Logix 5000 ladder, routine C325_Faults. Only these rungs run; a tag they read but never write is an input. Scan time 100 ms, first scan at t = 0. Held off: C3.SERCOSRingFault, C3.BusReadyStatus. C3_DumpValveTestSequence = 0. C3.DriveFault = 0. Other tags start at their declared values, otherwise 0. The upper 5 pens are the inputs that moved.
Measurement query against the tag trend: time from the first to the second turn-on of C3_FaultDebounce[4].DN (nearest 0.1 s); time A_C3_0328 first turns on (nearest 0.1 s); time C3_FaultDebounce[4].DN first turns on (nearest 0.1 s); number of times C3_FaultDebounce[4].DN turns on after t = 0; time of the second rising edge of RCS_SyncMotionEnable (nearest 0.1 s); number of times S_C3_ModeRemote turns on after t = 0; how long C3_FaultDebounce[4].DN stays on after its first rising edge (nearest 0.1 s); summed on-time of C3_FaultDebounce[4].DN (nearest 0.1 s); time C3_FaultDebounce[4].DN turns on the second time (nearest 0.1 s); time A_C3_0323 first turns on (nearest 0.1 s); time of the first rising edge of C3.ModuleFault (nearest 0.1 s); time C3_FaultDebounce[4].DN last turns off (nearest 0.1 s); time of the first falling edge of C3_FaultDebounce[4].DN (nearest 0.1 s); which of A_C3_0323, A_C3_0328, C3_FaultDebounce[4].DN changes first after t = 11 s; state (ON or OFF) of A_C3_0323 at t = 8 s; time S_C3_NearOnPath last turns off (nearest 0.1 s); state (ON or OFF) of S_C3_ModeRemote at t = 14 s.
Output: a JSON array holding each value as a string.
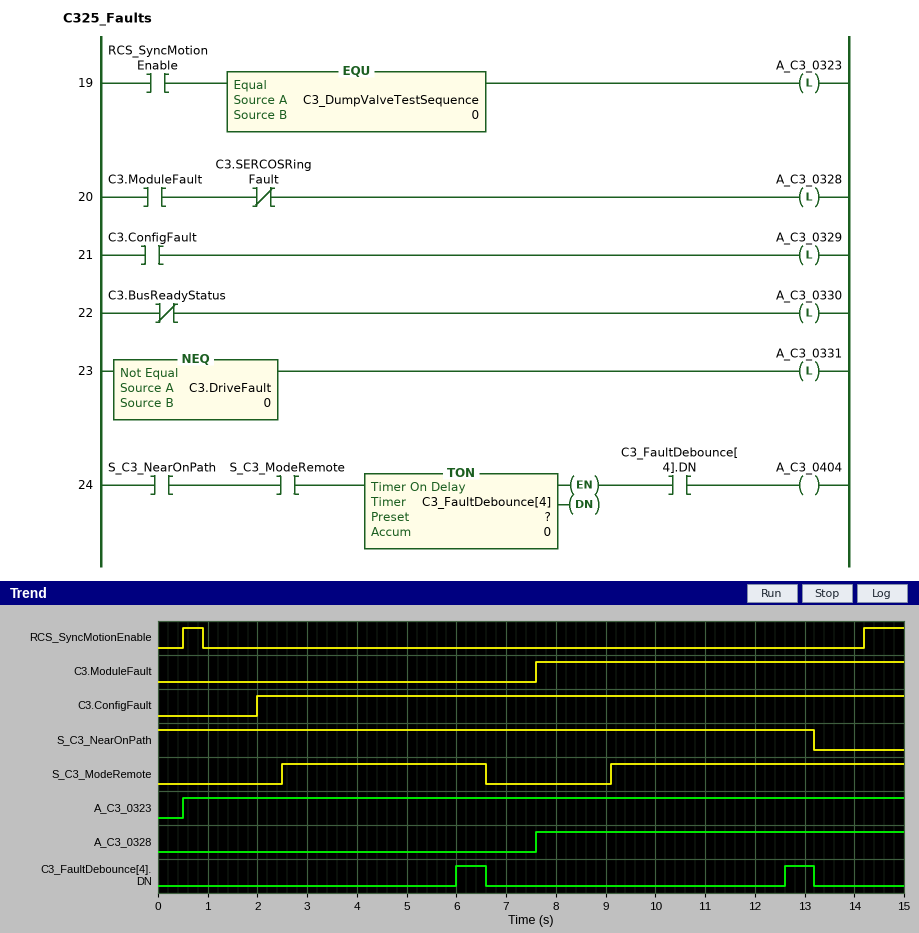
["6.6 s", "7.6 s", "6.0 s", "2", "14.2 s", "2", "0.6 s", "1.2 s", "12.6 s", "0.5 s", "7.6 s", "13.2 s", "6.6 s", "C3_FaultDebounce[4].DN", "ON", "13.2 s", "ON"]
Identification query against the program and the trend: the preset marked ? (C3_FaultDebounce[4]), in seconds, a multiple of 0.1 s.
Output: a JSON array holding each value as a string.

["3.5 s"]
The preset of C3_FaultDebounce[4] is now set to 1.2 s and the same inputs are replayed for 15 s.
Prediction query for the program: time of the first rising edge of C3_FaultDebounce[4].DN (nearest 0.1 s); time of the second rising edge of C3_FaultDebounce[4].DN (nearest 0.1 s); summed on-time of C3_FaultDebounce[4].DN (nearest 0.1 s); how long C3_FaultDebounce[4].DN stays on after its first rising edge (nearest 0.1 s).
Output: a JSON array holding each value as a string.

["3.7 s", "10.3 s", "5.8 s", "2.9 s"]
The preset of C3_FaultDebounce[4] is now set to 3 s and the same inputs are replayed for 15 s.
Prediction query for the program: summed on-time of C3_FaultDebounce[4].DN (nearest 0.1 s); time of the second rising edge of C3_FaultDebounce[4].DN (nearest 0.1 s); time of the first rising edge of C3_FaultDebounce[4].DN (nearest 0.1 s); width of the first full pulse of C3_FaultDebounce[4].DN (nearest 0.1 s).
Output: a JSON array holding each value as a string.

["2.2 s", "12.1 s", "5.5 s", "1.1 s"]
